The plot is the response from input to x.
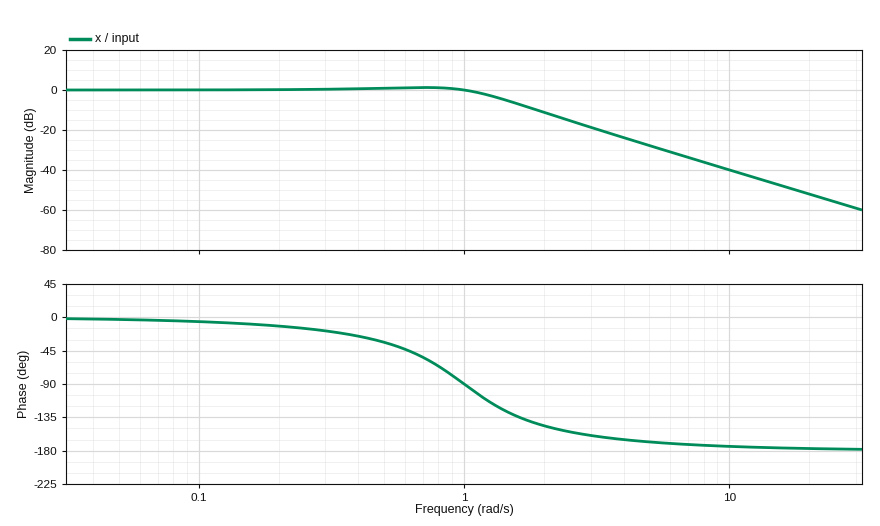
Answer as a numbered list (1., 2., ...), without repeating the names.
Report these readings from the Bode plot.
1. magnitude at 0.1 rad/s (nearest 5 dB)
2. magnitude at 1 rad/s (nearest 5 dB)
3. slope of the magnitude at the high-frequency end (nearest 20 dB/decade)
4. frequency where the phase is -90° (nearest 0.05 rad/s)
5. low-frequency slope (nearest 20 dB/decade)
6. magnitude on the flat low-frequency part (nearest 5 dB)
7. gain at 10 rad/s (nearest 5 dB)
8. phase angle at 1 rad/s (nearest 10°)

1. 0 dB
2. 0 dB
3. -40 dB/decade
4. 1.00 rad/s
5. 0 dB/decade
6. 0 dB
7. -40 dB
8. -90°
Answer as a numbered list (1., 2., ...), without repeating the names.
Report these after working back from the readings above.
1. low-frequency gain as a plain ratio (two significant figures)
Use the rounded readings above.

1. 1.0
